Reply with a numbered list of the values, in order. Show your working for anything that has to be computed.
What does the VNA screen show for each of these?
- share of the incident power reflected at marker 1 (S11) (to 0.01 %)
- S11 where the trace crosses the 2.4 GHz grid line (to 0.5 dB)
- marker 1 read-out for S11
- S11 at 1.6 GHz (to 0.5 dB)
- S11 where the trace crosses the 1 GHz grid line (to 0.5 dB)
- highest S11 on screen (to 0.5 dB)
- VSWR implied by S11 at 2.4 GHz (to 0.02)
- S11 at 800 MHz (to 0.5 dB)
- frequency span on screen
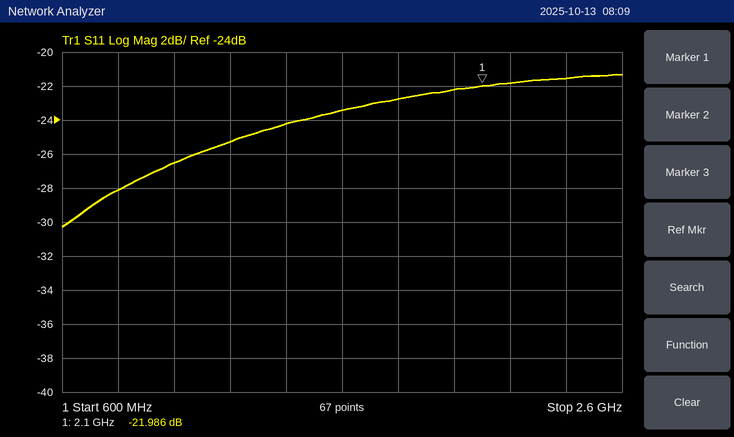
1. 10^(-21.986/10) ≈ 0.63 %
2. -21.5 dB
3. -21.986 dB
4. -23.5 dB
5. -26.5 dB
6. -21.5 dB
7. |Γ| = 10^(-21.5/20) = 0.0841; VSWR = (1 + 0.0841)/(1 − 0.0841) ≈ 1.18
8. -28.0 dB
9. 2 GHz
